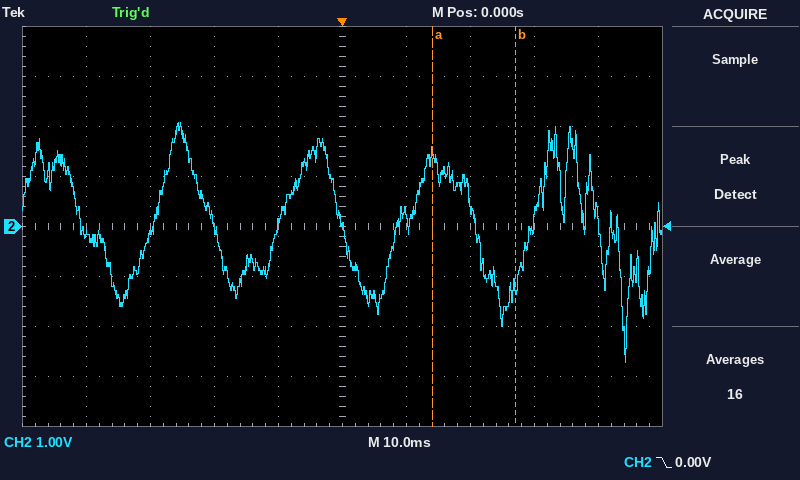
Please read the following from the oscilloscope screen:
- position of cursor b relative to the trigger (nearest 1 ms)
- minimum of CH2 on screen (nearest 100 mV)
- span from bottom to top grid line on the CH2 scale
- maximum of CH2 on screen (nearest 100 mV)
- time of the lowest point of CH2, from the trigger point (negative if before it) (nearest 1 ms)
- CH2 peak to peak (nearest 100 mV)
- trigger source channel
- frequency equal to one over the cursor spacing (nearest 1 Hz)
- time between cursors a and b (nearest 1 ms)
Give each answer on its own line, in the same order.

+27 ms
-2.7 V
8 V
2.1 V
+44 ms
4.8 V
CH2
77 Hz
13 ms
